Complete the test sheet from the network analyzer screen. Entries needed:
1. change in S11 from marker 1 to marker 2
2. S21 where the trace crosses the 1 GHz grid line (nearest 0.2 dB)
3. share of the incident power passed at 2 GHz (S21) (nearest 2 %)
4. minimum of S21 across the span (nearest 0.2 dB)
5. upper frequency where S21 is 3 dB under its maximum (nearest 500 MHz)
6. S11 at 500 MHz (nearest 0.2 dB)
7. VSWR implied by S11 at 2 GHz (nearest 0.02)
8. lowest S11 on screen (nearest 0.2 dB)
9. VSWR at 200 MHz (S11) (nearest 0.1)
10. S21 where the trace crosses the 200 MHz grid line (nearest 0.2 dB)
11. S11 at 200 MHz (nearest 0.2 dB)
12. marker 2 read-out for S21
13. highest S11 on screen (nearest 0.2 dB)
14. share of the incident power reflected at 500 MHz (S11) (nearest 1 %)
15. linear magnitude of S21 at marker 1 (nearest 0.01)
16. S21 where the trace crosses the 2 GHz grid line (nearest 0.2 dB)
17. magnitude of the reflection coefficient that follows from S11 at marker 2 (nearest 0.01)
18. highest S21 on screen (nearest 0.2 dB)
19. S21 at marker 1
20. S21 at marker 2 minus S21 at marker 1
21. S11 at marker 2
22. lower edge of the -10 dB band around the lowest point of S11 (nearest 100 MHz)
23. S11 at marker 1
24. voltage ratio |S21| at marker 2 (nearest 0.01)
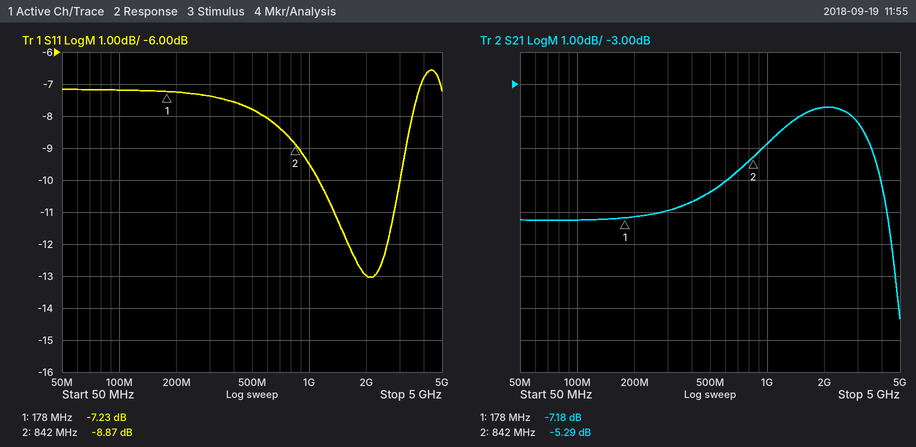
-1.64 dB
-4.8 dB
42 %
-10.4 dB
4.0 GHz
-7.8 dB
1.58
-13.0 dB
2.5
-7.2 dB
-7.2 dB
-5.29 dB
-6.6 dB
17 %
0.44
-3.8 dB
0.36
-3.8 dB
-7.18 dB
1.89 dB
-8.87 dB
1.1 GHz
-7.23 dB
0.54
